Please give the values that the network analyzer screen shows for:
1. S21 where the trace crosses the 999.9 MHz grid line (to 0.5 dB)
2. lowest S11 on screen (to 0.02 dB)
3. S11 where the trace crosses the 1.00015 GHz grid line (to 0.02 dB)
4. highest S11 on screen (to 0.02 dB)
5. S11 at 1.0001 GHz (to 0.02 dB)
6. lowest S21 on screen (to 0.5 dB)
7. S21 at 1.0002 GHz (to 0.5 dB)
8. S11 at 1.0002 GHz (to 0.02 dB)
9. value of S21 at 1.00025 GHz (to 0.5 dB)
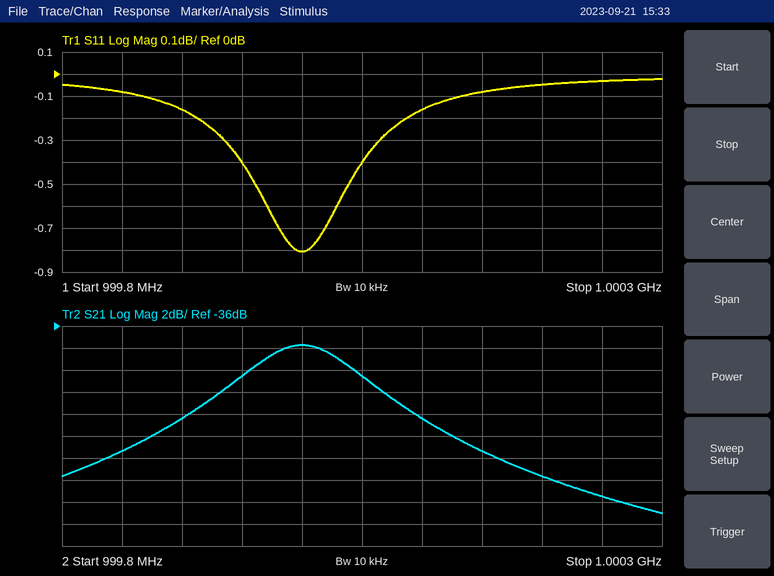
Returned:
-44.5 dB
-0.80 dB
-0.08 dB
-0.02 dB
-0.16 dB
-53.0 dB
-49.5 dB
-0.04 dB
-51.5 dB
